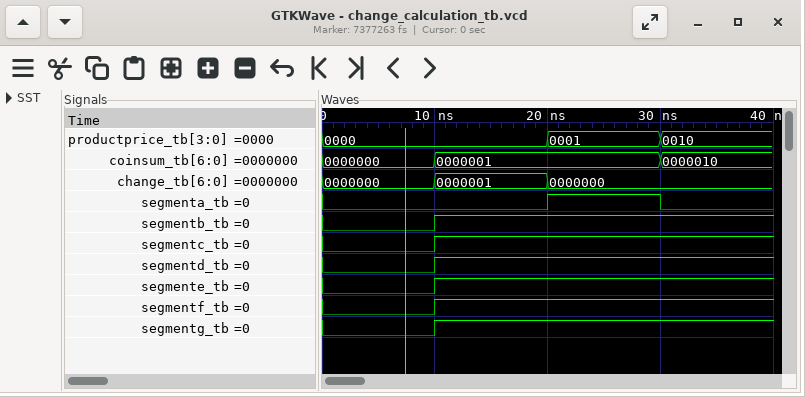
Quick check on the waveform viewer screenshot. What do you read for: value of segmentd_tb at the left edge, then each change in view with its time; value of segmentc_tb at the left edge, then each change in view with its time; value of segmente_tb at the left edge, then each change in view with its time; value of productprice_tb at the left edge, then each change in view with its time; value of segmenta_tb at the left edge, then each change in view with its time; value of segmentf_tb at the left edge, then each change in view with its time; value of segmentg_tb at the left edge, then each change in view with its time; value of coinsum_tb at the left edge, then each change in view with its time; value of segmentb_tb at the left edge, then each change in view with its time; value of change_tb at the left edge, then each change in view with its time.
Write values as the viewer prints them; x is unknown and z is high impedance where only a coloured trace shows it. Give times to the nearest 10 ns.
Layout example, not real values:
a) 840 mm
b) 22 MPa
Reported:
a) 0, 1 at 10 ns
b) 0, 1 at 10 ns
c) 0, 1 at 10 ns
d) 0000, 0001 at 20 ns, 0010 at 30 ns
e) 0, 1 at 20 ns, 0 at 30 ns
f) 0, 1 at 10 ns
g) 0, 1 at 10 ns
h) 0000000, 0000001 at 10 ns, 0000010 at 30 ns
i) 0, 1 at 10 ns
j) 0000000, 0000001 at 10 ns, 0000000 at 20 ns
